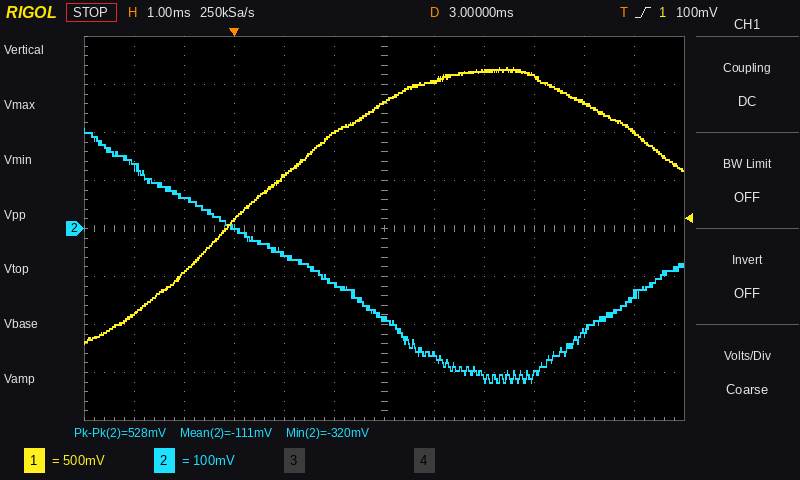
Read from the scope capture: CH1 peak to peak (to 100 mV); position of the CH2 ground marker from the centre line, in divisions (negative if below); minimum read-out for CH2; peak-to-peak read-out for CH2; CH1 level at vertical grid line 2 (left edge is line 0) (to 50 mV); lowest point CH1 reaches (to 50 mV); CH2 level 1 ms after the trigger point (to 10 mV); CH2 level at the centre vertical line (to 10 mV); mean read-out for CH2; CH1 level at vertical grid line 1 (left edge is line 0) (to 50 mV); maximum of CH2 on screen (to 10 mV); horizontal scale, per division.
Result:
2.90 V
0.0 div
-320 mV
528 mV
-450 mV
-1.20 V
-50 mV
-190 mV
-111 mV
-900 mV
210 mV
1 ms
